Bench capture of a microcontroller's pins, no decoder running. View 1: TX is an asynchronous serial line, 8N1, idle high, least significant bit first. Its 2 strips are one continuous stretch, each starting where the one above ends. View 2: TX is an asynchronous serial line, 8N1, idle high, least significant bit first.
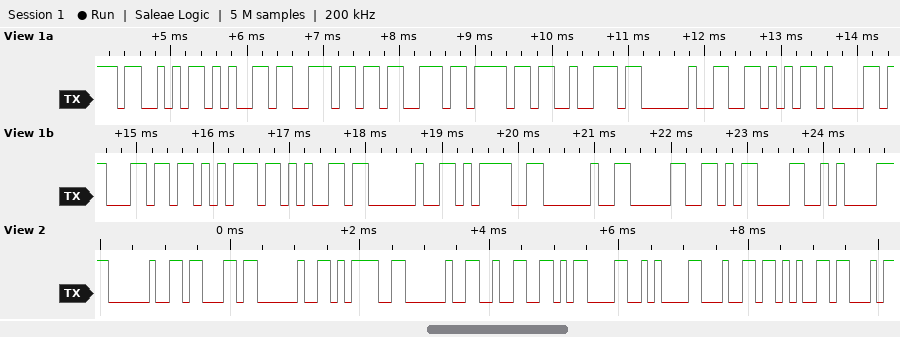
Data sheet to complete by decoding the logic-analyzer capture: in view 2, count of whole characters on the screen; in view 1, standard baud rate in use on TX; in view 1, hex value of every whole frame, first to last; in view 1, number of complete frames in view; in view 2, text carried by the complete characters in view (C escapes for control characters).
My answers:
10
9600 baud
53 65 6E 73 6F 72 20 56 61 6C 75 65 20 3D 20 30 0D 0A
18
" c = 2\r\nde"
